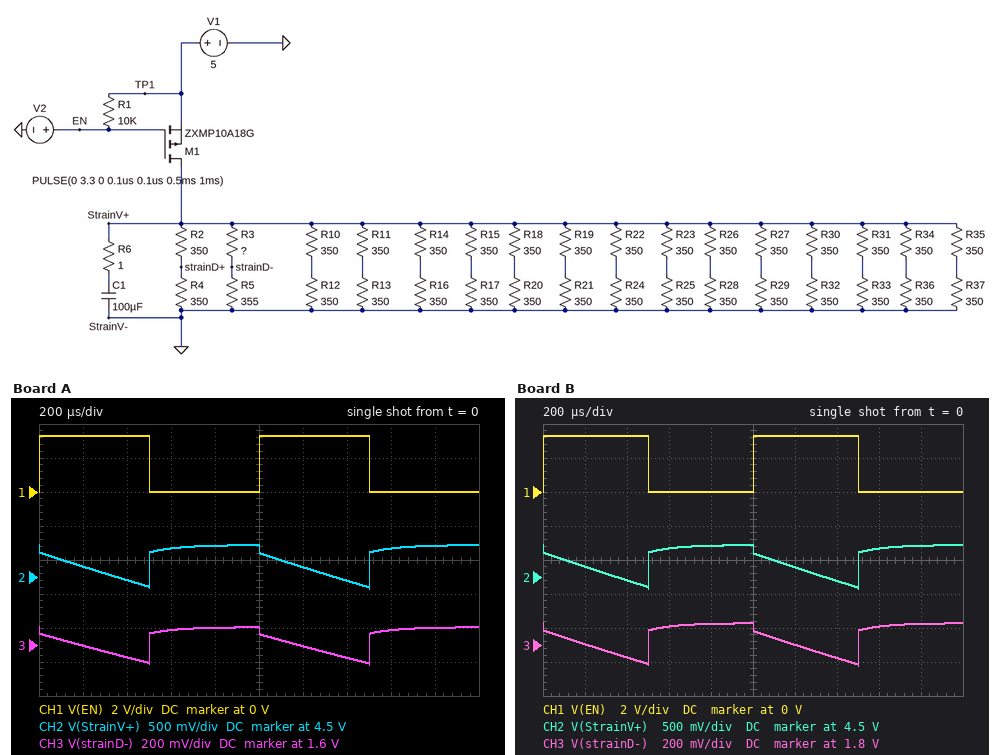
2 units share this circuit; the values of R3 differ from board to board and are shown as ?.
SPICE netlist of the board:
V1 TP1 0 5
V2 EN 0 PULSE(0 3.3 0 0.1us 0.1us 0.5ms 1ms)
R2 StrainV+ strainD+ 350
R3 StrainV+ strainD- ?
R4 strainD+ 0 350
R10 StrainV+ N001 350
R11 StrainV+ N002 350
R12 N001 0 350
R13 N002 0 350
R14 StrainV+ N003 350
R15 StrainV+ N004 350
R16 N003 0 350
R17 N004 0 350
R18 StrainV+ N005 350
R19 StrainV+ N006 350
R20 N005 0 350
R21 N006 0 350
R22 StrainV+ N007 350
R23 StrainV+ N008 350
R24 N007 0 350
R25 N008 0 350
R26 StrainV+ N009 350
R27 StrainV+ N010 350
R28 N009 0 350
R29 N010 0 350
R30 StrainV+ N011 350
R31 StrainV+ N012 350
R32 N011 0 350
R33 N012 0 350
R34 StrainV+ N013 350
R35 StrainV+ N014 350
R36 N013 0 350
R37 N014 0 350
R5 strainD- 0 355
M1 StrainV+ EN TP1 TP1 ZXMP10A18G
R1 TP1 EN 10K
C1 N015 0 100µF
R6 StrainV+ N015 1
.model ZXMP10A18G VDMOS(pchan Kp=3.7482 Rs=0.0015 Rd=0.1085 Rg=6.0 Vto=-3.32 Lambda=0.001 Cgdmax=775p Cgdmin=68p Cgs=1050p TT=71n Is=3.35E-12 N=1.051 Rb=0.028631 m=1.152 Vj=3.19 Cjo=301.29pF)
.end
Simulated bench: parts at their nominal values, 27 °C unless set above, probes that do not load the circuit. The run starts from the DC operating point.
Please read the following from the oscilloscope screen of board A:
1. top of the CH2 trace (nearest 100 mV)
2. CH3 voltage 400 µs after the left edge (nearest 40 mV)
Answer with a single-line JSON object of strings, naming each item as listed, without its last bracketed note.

{"top of the CH2 trace": "5.0 V", "CH3 voltage 400 µs after the left edge": "1.52 V"}
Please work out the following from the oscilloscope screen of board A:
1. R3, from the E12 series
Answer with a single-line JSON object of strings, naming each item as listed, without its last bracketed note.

{"R3, from the E12 series": "680 Ω"}
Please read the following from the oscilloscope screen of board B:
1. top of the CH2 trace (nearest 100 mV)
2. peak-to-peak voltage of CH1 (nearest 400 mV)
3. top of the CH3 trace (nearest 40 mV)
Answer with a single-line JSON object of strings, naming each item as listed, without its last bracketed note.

{"top of the CH2 trace": "5.0 V", "peak-to-peak voltage of CH1": "3.2 V", "top of the CH3 trace": "1.92 V"}
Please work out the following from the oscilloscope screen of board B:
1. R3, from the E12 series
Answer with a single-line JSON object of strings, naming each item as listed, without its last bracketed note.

{"R3, from the E12 series": "560 Ω"}
